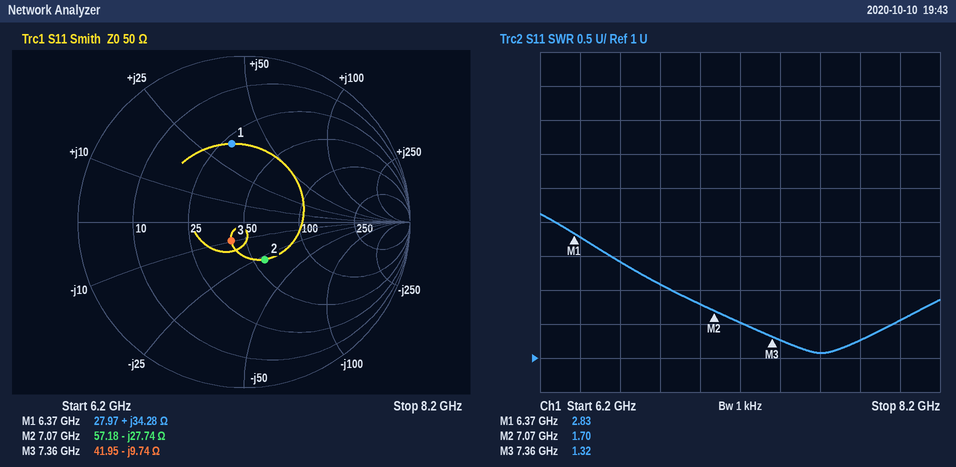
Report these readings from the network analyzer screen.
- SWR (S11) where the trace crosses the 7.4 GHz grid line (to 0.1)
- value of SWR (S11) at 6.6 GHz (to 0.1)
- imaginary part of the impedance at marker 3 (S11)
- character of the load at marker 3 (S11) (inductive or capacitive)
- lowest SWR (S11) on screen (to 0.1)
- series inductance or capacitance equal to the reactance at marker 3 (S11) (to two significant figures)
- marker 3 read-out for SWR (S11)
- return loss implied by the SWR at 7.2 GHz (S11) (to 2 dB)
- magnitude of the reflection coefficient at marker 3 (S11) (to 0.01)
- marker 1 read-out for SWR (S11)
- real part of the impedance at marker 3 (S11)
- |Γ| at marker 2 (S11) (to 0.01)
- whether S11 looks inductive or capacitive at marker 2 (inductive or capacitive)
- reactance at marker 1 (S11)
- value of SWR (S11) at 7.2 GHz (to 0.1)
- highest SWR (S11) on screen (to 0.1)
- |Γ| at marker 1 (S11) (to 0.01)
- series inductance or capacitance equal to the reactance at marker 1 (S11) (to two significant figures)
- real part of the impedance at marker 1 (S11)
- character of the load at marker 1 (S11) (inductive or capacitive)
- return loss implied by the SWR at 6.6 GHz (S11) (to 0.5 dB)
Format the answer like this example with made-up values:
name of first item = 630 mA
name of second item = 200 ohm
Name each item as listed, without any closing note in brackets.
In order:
SWR (S11) where the trace crosses the 7.4 GHz grid line = 1.3
value of SWR (S11) at 6.6 GHz = 2.4
imaginary part of the impedance at marker 3 = -9.74 Ω
character of the load at marker 3 (S11) = capacitive
lowest SWR (S11) on screen = 1.1
series inductance or capacitance equal to the reactance at marker 3 (S11) = 2.2 pF
marker 3 read-out for SWR = 1.32
return loss implied by the SWR at 7.2 GHz (S11) = 14 dB
magnitude of the reflection coefficient at marker 3 (S11) = 0.14
marker 1 read-out for SWR = 2.83
real part of the impedance at marker 3 = 41.95 Ω
|Γ| at marker 2 (S11) = 0.26
whether S11 looks inductive or capacitive at marker 2 = capacitive
reactance at marker 1 = +34.28 Ω
value of SWR (S11) at 7.2 GHz = 1.5
highest SWR (S11) on screen = 3.1
|Γ| at marker 1 (S11) = 0.48
series inductance or capacitance equal to the reactance at marker 1 (S11) = 860 pH
real part of the impedance at marker 1 = 27.97 Ω
character of the load at marker 1 (S11) = inductive
return loss implied by the SWR at 6.6 GHz (S11) = 7.5 dB
